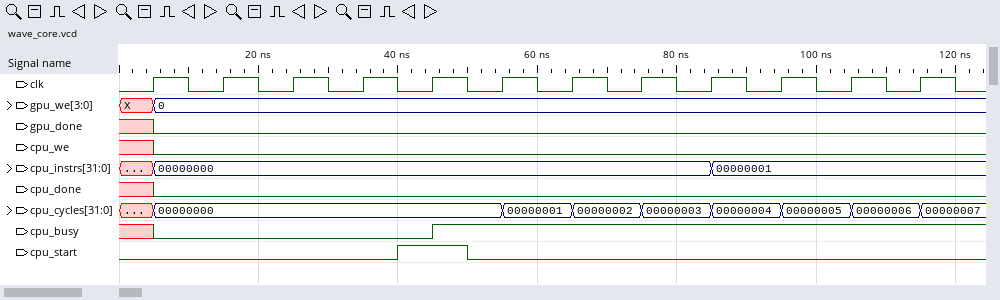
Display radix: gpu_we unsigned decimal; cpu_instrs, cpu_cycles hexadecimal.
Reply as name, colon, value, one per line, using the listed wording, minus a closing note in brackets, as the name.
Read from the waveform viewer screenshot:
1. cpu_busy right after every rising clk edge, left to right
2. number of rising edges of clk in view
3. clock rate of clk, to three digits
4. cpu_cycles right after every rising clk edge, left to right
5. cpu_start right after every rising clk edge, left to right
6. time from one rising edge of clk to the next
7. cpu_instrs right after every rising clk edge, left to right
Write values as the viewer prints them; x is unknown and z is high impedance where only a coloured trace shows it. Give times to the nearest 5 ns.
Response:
cpu_busy right after every rising clk edge, left to right: 0 0 0 0 1 1 1 1 1 1 1 1
number of rising edges of clk in view: 12
clock rate of clk, to three digits: 100 MHz
cpu_cycles right after every rising clk edge, left to right: 00000000, 00000000, 00000000, 00000000, 00000000, 00000001, 00000002, 00000003, 00000004, 00000005, 00000006, 00000007
cpu_start right after every rising clk edge, left to right: 0 0 0 0 1 0 0 0 0 0 0 0
time from one rising edge of clk to the next: 10 ns
cpu_instrs right after every rising clk edge, left to right: 00000000, 00000000, 00000000, 00000000, 00000000, 00000000, 00000000, 00000000, 00000001, 00000001, 00000001, 00000001
